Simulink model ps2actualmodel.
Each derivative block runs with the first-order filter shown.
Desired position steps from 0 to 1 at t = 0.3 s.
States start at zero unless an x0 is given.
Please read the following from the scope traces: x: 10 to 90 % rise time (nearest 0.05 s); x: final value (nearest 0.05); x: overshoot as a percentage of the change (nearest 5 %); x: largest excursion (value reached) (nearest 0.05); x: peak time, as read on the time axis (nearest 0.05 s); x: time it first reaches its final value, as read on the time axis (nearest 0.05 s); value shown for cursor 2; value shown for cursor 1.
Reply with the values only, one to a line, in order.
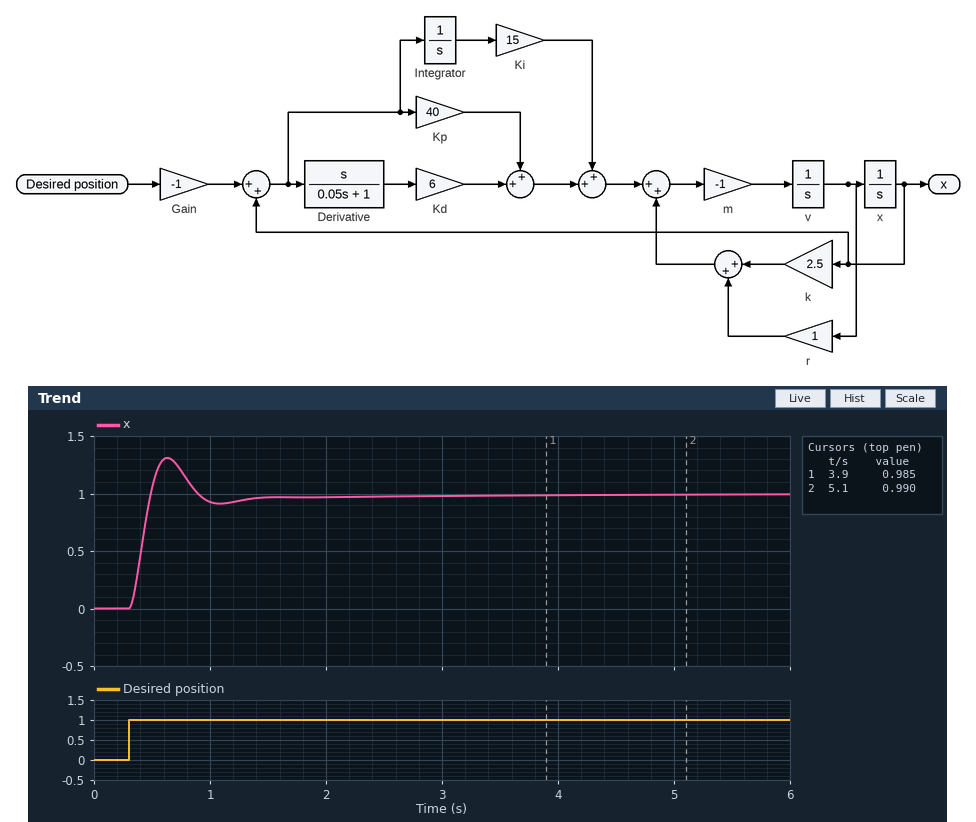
0.15 s
1.00
30 %
1.30
0.65 s
0.50 s
0.990
0.985
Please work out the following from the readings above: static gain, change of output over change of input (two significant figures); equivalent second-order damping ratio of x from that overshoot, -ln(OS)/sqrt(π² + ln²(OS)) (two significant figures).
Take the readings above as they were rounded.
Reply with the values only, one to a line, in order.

1.0
0.36
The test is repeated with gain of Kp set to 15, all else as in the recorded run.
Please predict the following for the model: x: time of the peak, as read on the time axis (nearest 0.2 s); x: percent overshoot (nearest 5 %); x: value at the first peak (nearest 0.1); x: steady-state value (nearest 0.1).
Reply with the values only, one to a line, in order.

0.8 s
10 %
1.1
1.0
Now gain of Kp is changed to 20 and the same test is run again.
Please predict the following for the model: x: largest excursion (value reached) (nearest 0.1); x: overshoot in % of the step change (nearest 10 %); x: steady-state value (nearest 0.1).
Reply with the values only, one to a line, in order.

1.2
20 %
1.0
